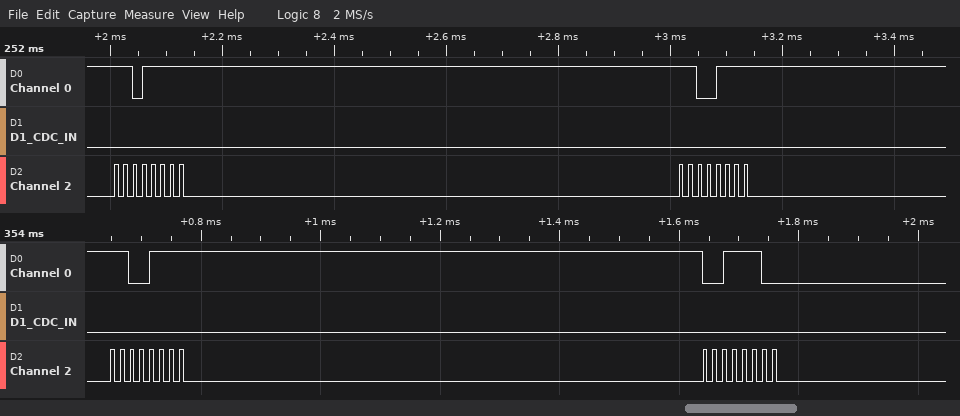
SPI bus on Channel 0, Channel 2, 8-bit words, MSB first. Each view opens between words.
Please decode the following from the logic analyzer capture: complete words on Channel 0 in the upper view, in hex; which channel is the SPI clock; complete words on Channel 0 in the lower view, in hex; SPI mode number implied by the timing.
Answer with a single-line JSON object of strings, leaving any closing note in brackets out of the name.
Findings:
{"complete words on Channel 0 in the upper view, in hex": "DF, CF", "which channel is the SPI clock": "Channel 2", "complete words on Channel 0 in the lower view, in hex": "CF, 3C", "SPI mode number implied by the timing": "1"}
